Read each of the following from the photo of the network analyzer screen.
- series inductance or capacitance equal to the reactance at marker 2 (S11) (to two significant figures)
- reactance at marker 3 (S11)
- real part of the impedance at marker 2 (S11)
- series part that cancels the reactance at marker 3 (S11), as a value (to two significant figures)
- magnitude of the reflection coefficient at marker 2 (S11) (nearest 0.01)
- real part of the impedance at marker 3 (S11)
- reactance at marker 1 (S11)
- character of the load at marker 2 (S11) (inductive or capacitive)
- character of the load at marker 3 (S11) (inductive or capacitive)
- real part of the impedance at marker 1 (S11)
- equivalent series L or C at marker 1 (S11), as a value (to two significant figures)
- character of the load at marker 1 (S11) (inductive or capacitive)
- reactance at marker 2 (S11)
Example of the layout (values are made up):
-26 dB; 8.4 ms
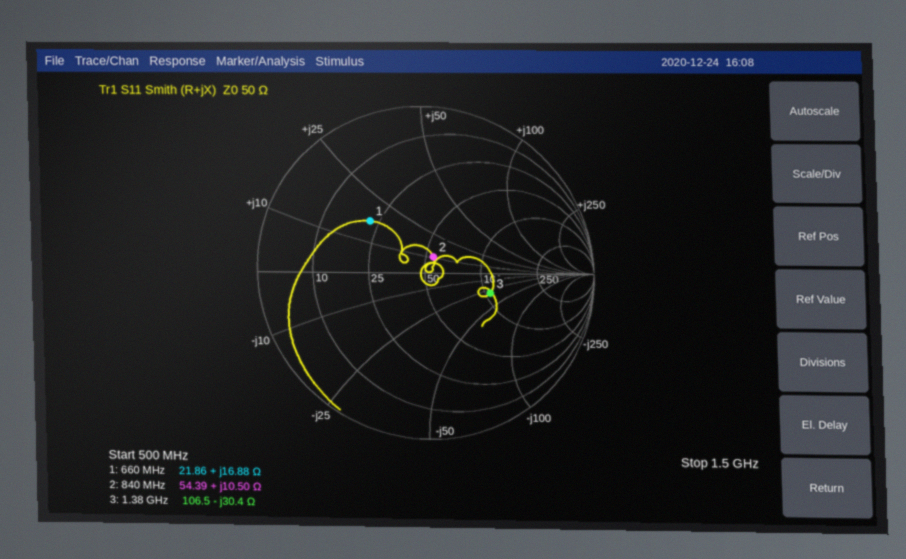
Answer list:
2.0 nH; -30.4 Ω; 54.39 Ω; 3.5 nH; 0.11; 106.5 Ω; +16.88 Ω; inductive; capacitive; 21.86 Ω; 4.1 nH; inductive; +10.50 Ω
